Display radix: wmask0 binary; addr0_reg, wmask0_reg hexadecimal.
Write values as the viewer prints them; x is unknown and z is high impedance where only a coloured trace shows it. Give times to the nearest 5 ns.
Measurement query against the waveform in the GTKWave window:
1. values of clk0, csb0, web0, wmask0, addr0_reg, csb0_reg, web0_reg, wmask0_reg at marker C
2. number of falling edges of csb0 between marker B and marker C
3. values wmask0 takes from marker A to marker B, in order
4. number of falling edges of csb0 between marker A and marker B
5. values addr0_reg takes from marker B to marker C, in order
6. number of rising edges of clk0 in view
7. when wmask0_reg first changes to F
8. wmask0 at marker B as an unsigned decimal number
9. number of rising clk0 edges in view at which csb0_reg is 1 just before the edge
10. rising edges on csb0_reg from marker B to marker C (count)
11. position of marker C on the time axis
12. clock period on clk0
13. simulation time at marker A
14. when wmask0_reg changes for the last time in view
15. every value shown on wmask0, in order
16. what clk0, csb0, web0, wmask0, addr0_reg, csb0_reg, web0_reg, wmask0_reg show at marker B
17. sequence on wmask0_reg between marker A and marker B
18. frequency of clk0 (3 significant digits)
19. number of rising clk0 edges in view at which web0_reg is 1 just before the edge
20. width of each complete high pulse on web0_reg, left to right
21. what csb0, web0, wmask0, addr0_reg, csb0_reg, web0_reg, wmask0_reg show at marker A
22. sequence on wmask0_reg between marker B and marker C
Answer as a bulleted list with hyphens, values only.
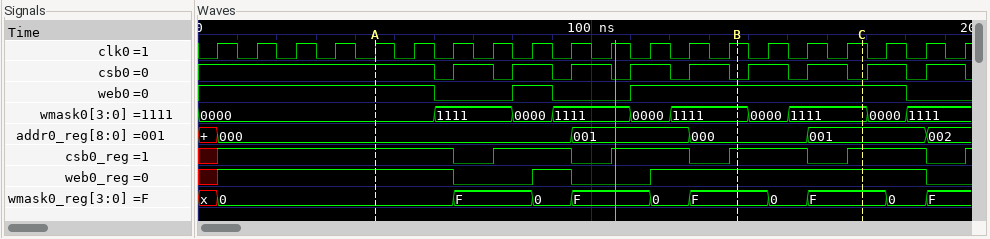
- clk0=1, csb0=0, web0=1, wmask0=1111, addr0_reg=001, csb0_reg=1, web0_reg=1, wmask0_reg=F
- 2
- 0000, 1111, 0000, 1111, 0000, 1111
- 6
- 000, 001
- 20
- 65 ns
- 15
- 14
- 1
- 170 ns
- 10 ns
- 45 ns
- 185 ns
- 0000, 1111, 0000, 1111, 0000, 1111, 0000, 1111, 0000, 1111
- clk0=1, csb0=0, web0=1, wmask0=1111, addr0_reg=000, csb0_reg=1, web0_reg=1, wmask0_reg=F
- 0, F, 0, F, 0, F
- 100 MHz
- 14
- 10 ns, 70 ns
- csb0=1, web0=1, wmask0=0000, addr0_reg=000, csb0_reg=1, web0_reg=1, wmask0_reg=0
- F, 0, F
